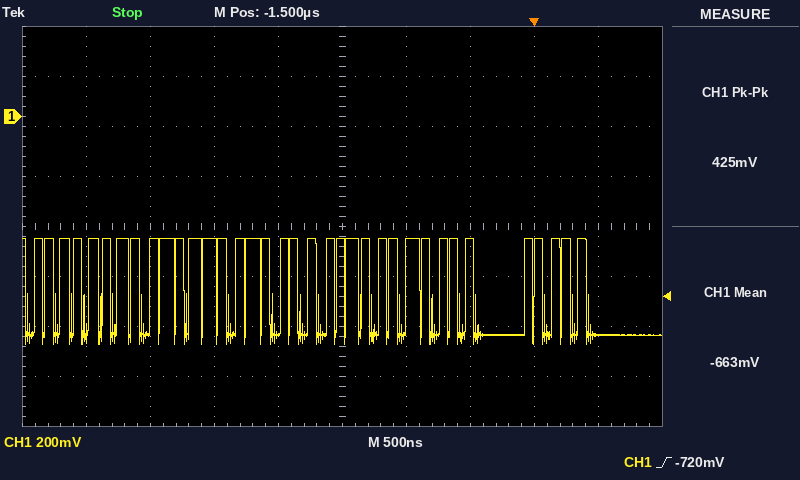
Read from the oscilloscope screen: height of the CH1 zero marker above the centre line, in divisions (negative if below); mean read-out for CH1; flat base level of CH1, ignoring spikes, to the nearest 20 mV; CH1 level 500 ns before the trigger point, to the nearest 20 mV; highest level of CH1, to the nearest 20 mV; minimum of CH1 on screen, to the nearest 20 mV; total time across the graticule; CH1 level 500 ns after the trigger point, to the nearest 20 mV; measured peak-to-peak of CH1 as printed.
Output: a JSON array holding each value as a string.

["+2.2 div", "-663 mV", "-880 mV", "-480 mV", "-480 mV", "-920 mV", "5 µs", "-880 mV", "425 mV"]
